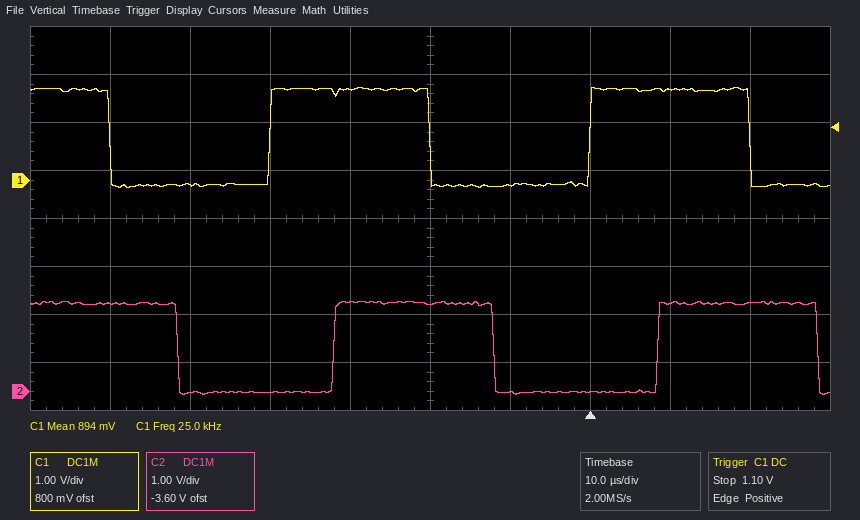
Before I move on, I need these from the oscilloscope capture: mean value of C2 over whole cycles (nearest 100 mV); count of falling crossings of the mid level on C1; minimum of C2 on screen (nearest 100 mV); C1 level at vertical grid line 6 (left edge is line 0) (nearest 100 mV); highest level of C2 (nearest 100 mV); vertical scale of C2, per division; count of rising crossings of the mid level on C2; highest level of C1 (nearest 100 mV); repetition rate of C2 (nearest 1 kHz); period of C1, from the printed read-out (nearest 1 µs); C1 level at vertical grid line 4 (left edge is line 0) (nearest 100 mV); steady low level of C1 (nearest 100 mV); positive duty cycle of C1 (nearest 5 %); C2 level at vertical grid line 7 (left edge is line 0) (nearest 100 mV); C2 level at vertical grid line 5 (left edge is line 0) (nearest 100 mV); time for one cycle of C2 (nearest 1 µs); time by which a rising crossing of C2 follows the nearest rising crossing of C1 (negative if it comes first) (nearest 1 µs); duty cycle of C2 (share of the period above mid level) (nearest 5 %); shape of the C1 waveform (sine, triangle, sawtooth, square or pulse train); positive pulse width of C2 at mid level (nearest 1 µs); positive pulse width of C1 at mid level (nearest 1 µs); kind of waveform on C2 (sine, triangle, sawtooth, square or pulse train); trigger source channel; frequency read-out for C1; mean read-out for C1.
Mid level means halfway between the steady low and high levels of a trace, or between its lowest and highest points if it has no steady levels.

900 mV
3
-100 mV
-100 mV
1.9 V
1 V
2
1.9 V
25 kHz
40 µs
1.9 V
-100 mV
50 %
0.0 V
1.8 V
40 µs
+8 µs
50 %
square
20 µs
20 µs
square
C1
25.0 kHz
894 mV
